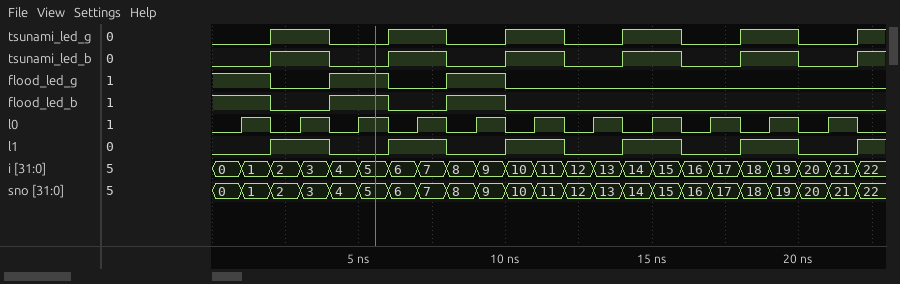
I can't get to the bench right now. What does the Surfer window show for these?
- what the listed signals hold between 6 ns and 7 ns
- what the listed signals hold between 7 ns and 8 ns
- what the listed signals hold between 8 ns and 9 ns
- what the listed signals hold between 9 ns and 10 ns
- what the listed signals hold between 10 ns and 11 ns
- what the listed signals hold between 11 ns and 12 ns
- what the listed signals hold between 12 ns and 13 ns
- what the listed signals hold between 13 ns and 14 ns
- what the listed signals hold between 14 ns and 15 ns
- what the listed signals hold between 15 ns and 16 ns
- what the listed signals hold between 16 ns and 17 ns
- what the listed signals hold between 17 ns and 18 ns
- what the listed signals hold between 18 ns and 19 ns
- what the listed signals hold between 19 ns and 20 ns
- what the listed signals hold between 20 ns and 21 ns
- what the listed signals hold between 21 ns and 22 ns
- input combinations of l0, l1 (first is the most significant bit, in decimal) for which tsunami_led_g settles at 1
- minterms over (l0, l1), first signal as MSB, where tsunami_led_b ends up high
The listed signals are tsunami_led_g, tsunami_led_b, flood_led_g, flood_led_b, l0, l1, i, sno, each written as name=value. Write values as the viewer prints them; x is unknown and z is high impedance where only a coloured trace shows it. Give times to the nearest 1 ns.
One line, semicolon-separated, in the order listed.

tsunami_led_g=1, tsunami_led_b=1, flood_led_g=0, flood_led_b=0, l0=0, l1=1, i=6, sno=6; tsunami_led_g=1, tsunami_led_b=1, flood_led_g=0, flood_led_b=0, l0=1, l1=1, i=7, sno=7; tsunami_led_g=0, tsunami_led_b=0, flood_led_g=1, flood_led_b=1, l0=0, l1=0, i=8, sno=8; tsunami_led_g=0, tsunami_led_b=0, flood_led_g=1, flood_led_b=1, l0=1, l1=0, i=9, sno=9; tsunami_led_g=1, tsunami_led_b=1, flood_led_g=0, flood_led_b=0, l0=0, l1=1, i=10, sno=10; tsunami_led_g=1, tsunami_led_b=1, flood_led_g=0, flood_led_b=0, l0=1, l1=1, i=11, sno=11; tsunami_led_g=0, tsunami_led_b=0, flood_led_g=0, flood_led_b=0, l0=0, l1=0, i=12, sno=12; tsunami_led_g=0, tsunami_led_b=0, flood_led_g=0, flood_led_b=0, l0=1, l1=0, i=13, sno=13; tsunami_led_g=1, tsunami_led_b=1, flood_led_g=0, flood_led_b=0, l0=0, l1=1, i=14, sno=14; tsunami_led_g=1, tsunami_led_b=1, flood_led_g=0, flood_led_b=0, l0=1, l1=1, i=15, sno=15; tsunami_led_g=0, tsunami_led_b=0, flood_led_g=0, flood_led_b=0, l0=0, l1=0, i=16, sno=16; tsunami_led_g=0, tsunami_led_b=0, flood_led_g=0, flood_led_b=0, l0=1, l1=0, i=17, sno=17; tsunami_led_g=1, tsunami_led_b=1, flood_led_g=0, flood_led_b=0, l0=0, l1=1, i=18, sno=18; tsunami_led_g=1, tsunami_led_b=1, flood_led_g=0, flood_led_b=0, l0=1, l1=1, i=19, sno=19; tsunami_led_g=0, tsunami_led_b=0, flood_led_g=0, flood_led_b=0, l0=0, l1=0, i=20, sno=20; tsunami_led_g=0, tsunami_led_b=0, flood_led_g=0, flood_led_b=0, l0=1, l1=0, i=21, sno=21; 1, 3; 1, 3
